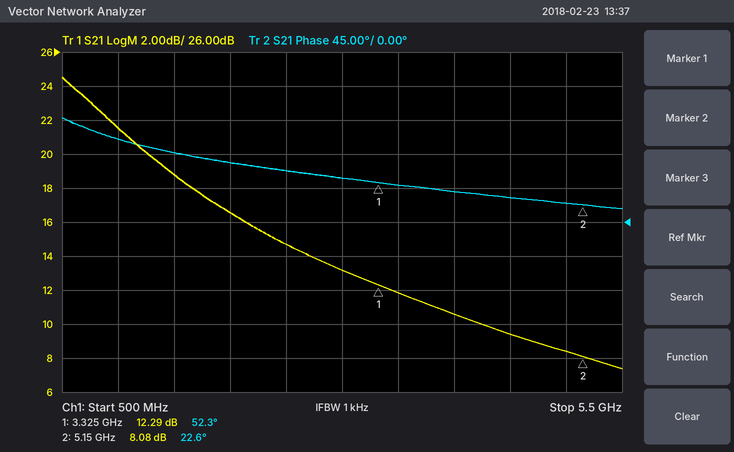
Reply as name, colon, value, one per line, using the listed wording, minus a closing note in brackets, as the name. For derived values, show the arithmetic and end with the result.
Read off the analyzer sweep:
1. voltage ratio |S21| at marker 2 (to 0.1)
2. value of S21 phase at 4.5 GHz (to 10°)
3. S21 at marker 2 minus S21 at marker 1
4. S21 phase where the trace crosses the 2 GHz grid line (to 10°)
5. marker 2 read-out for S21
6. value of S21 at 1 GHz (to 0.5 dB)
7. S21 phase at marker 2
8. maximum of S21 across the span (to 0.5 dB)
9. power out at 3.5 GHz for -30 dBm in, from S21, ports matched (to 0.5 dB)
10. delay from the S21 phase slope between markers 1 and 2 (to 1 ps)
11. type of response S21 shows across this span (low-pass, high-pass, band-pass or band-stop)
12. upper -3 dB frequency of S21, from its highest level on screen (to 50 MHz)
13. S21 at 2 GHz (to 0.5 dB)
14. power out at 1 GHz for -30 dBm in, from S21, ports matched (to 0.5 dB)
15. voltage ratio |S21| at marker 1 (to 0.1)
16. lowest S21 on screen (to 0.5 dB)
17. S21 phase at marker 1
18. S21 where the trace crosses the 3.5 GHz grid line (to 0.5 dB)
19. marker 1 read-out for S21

voltage ratio |S21| at marker 2: 10^(8.08/20) ≈ 2.5
value of S21 phase at 4.5 GHz: 30°
S21 at marker 2 minus S21 at marker 1: 8.08 − (12.29) = -4.21 dB
S21 phase where the trace crosses the 2 GHz grid line: 80°
marker 2 read-out for S21: 8.08 dB
value of S21 at 1 GHz: 21.5 dB
S21 phase at marker 2: 22.6°
maximum of S21 across the span: 24.5 dB
power out at 3.5 GHz for -30 dBm in, from S21, ports matched: -30 dBm + (12.0 dB) = -18.0 dBm
delay from the S21 phase slope between markers 1 and 2: −(22.6° − (52.3°))/(360° × 1.825 GHz) ≈ 45 ps
type of response S21 shows across this span: low-pass
upper -3 dB frequency of S21, from its highest level on screen: 1.00 GHz
S21 at 2 GHz: 16.5 dB
power out at 1 GHz for -30 dBm in, from S21, ports matched: -30 dBm + (21.5 dB) = -8.5 dBm
voltage ratio |S21| at marker 1: 10^(12.29/20) ≈ 4.1
lowest S21 on screen: 7.5 dB
S21 phase at marker 1: 52.3°
S21 where the trace crosses the 3.5 GHz grid line: 12.0 dB
marker 1 read-out for S21: 12.29 dB
